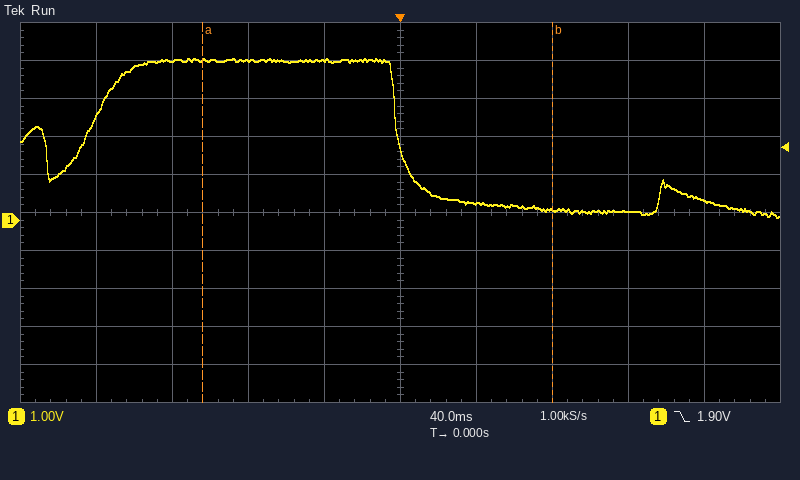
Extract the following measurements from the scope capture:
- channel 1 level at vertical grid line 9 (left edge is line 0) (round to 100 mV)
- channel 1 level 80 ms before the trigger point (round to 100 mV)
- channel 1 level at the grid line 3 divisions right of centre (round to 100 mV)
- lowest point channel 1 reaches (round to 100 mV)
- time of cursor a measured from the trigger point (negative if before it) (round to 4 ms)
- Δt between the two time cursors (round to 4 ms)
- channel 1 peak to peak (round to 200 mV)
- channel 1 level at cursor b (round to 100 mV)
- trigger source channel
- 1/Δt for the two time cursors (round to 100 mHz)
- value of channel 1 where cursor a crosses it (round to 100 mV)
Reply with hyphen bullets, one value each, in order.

- 500 mV
- 4.2 V
- 200 mV
- 100 mV
- -104 ms
- 184 ms
- 4.2 V
- 300 mV
- channel 1
- 5.4 Hz
- 4.2 V
